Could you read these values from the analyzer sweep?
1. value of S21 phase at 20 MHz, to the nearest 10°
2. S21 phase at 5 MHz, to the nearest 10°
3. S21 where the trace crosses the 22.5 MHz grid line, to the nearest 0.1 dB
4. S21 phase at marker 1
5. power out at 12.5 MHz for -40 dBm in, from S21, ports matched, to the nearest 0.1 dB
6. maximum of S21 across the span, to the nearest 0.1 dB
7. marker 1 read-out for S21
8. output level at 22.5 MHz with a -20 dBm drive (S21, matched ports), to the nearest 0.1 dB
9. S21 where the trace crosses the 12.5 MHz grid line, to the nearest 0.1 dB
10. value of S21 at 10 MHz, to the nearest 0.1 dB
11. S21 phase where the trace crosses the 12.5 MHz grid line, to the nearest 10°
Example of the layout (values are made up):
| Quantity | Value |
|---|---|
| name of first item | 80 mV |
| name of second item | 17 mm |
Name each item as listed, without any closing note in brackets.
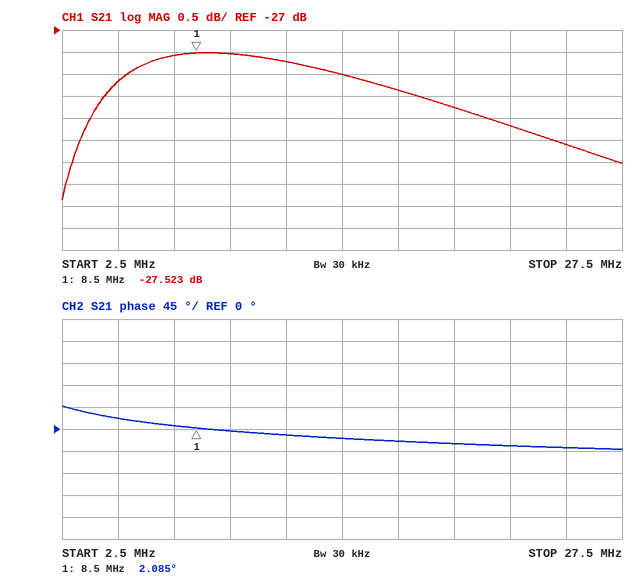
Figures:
| Quantity | Value |
|---|---|
| value of S21 phase at 20 MHz, to the nearest 10° | -30° |
| S21 phase at 5 MHz, to the nearest 10° | 20° |
| S21 where the trace crosses the 22.5 MHz grid line, to the nearest 0.1 dB | -29.2 dB |
| S21 phase at marker 1 | 2.085° |
| power out at 12.5 MHz for -40 dBm in, from S21, ports matched, to the nearest 0.1 dB | -67.7 dBm |
| maximum of S21 across the span, to the nearest 0.1 dB | -27.5 dB |
| marker 1 read-out for S21 | -27.523 dB |
| output level at 22.5 MHz with a -20 dBm drive (S21, matched ports), to the nearest 0.1 dB | -49.2 dBm |
| S21 where the trace crosses the 12.5 MHz grid line, to the nearest 0.1 dB | -27.7 dB |
| value of S21 at 10 MHz, to the nearest 0.1 dB | -27.5 dB |
| S21 phase where the trace crosses the 12.5 MHz grid line, to the nearest 10° | -10° |
